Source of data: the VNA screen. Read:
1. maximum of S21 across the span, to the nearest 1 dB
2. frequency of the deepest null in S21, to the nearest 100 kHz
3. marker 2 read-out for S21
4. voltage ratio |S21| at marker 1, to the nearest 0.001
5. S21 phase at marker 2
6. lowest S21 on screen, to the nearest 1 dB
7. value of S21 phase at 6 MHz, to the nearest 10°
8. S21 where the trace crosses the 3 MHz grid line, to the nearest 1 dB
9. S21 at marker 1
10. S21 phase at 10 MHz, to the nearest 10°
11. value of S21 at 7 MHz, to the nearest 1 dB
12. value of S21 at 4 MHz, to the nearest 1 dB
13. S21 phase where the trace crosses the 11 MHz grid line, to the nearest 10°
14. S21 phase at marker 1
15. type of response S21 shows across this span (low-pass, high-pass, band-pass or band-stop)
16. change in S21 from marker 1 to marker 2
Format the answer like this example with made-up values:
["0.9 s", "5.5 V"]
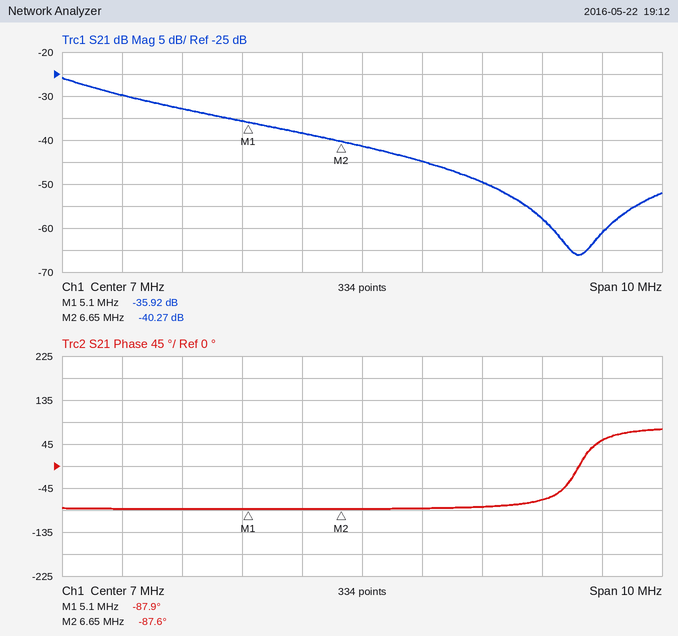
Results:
["-26 dB", "10.6 MHz", "-40.27 dB", "0.016", "-87.6°", "-66 dB", "-90°", "-30 dB", "-35.92 dB", "-70°", "-41 dB", "-33 dB", "50°", "-87.9°", "low-pass", "-4.35 dB"]
